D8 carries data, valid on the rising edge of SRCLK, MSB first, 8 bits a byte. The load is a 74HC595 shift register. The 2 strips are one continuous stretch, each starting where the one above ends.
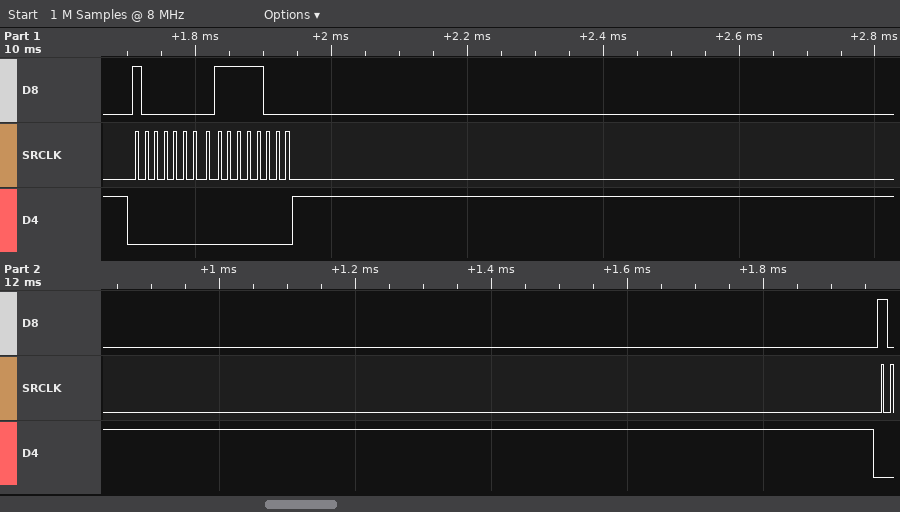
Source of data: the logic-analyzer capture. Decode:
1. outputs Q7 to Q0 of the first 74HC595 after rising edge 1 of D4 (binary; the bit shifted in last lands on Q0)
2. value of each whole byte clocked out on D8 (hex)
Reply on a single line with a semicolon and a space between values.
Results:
11111000; 80 F8
